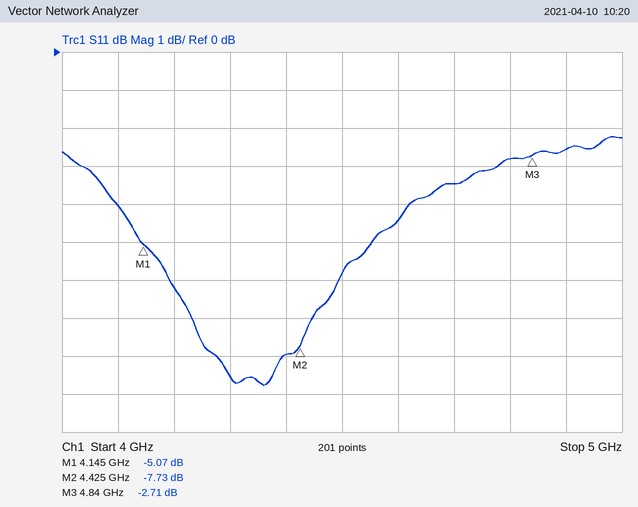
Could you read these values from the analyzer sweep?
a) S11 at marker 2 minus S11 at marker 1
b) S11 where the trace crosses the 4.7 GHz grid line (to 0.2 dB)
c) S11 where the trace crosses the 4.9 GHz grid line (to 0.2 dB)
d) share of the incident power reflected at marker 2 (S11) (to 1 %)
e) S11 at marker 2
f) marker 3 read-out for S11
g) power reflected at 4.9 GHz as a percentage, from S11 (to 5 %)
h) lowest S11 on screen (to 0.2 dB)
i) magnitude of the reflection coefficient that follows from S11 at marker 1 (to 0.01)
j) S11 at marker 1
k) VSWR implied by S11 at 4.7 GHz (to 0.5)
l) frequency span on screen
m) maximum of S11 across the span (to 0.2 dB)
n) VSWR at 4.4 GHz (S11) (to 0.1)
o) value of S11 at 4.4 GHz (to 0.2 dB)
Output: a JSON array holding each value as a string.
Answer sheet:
["-2.66 dB", "-3.4 dB", "-2.6 dB", "17 %", "-7.73 dB", "-2.71 dB", "55 %", "-8.8 dB", "0.56", "-5.07 dB", "5.0", "1 GHz", "-2.2 dB", "2.3", "-8.0 dB"]
